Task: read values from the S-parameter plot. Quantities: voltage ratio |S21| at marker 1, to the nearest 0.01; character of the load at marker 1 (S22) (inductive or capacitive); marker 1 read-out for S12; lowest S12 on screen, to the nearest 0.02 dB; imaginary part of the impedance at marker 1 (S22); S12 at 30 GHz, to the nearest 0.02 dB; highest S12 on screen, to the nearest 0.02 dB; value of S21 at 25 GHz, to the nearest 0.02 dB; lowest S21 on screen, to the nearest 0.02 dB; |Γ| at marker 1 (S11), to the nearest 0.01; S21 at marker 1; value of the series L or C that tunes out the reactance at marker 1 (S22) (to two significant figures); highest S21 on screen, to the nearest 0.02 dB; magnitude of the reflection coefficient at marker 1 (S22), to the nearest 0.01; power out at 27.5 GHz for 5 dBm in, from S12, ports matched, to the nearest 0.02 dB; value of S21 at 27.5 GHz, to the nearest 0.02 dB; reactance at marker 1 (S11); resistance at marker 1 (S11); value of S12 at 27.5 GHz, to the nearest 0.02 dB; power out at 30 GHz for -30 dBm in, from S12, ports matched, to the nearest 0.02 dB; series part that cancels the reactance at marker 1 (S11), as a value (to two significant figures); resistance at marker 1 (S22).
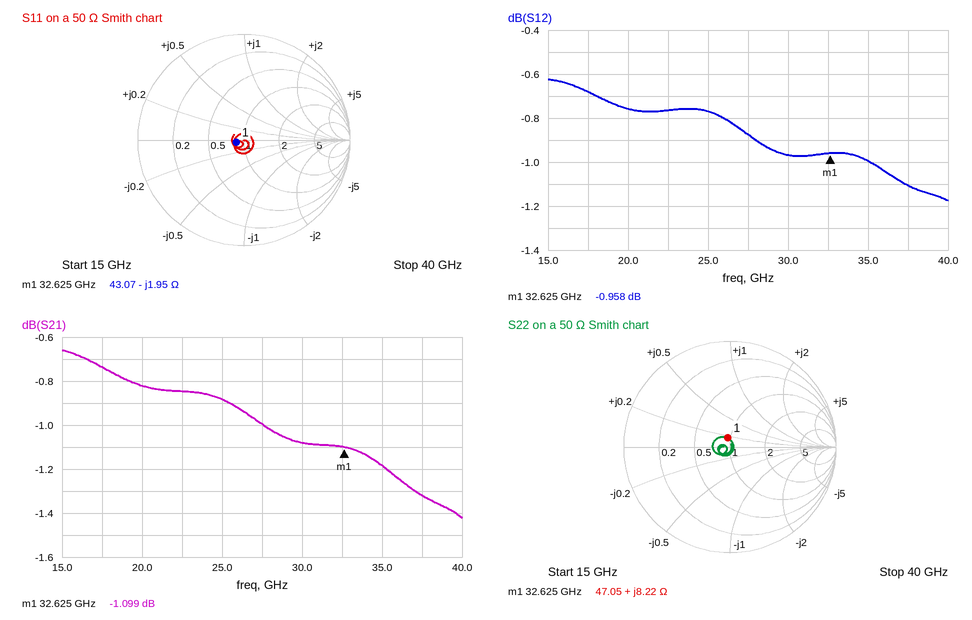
0.88
inductive
-0.958 dB
-1.18 dB
+8.22 Ω
-0.96 dB
-0.62 dB
-0.88 dB
-1.42 dB
0.08
-1.099 dB
590 fF
-0.66 dB
0.09
4.12 dBm
-1.00 dB
-1.95 Ω
43.07 Ω
-0.88 dB
-30.96 dBm
9.5 pH
47.05 Ω
